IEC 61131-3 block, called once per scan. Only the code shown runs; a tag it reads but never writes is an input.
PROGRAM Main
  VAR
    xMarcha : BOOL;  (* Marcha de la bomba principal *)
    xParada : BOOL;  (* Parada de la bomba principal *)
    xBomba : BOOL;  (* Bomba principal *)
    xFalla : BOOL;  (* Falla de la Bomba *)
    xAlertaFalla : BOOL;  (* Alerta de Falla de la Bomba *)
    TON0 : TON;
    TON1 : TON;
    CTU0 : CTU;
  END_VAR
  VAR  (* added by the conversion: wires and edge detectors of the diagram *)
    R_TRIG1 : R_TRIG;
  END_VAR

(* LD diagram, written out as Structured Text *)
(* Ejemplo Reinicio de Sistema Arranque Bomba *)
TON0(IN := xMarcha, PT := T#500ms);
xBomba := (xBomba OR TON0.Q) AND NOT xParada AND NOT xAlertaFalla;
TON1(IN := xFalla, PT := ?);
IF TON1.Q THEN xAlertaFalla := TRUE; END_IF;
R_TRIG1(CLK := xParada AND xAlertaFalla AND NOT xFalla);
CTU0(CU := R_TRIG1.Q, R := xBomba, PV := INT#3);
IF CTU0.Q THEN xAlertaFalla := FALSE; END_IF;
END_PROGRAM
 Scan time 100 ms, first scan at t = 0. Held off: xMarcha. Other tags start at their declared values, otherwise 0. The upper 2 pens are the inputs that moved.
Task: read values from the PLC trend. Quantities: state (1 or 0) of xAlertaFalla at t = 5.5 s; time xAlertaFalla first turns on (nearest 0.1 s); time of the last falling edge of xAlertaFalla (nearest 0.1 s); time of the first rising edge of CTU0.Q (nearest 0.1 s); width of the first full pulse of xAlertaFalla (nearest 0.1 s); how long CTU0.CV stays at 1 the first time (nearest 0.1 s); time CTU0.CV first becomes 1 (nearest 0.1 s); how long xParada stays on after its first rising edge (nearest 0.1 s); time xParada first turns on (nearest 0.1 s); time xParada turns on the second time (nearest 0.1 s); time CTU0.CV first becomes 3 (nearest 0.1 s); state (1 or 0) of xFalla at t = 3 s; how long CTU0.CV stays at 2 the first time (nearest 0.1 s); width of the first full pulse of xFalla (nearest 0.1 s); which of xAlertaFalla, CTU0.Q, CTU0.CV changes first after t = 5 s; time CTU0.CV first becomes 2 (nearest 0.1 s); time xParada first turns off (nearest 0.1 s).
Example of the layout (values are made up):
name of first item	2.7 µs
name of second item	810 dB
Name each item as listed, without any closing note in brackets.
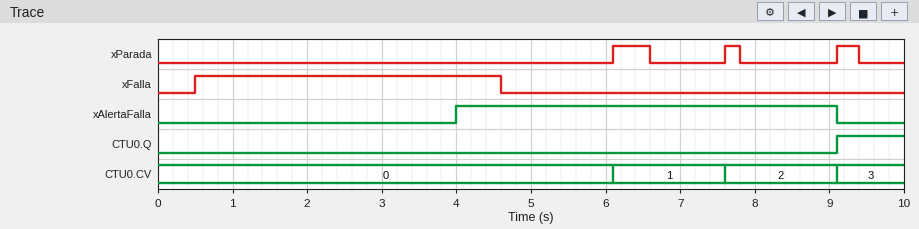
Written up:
state (1 or 0) of xAlertaFalla at t = 5.5 s	1
time xAlertaFalla first turns on	4.0 s
time of the last falling edge of xAlertaFalla	9.1 s
time of the first rising edge of CTU0.Q	9.1 s
width of the first full pulse of xAlertaFalla	5.1 s
how long CTU0.CV stays at 1 the first time	1.5 s
time CTU0.CV first becomes 1	6.1 s
how long xParada stays on after its first rising edge	0.5 s
time xParada first turns on	6.1 s
time xParada turns on the second time	7.6 s
time CTU0.CV first becomes 3	9.1 s
state (1 or 0) of xFalla at t = 3 s	1
how long CTU0.CV stays at 2 the first time	1.5 s
width of the first full pulse of xFalla	4.1 s
which of xAlertaFalla, CTU0.Q, CTU0.CV changes first after t = 5 s	CTU0.CV
time CTU0.CV first becomes 2	7.6 s
time xParada first turns off	6.6 s
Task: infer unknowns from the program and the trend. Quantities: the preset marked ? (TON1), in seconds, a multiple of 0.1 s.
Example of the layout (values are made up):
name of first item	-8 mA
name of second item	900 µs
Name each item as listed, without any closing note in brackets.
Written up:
the preset marked ? (TON1), in seconds, a multiple of 0.1 s	3.5 s
